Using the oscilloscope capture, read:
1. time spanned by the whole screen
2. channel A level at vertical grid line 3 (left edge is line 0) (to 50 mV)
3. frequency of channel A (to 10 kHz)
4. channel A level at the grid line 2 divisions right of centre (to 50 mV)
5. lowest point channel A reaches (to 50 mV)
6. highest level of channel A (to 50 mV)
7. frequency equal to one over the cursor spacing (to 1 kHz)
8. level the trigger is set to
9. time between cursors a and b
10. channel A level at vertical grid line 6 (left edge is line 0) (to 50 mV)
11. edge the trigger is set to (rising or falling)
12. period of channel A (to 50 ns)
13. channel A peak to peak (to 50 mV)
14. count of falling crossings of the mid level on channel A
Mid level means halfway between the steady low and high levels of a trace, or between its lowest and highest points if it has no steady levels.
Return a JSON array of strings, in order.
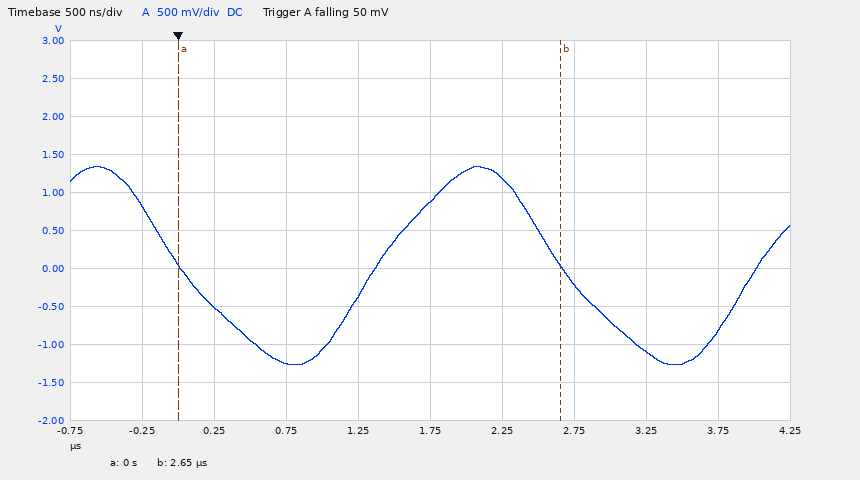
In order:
["5 µs", "-1.25 V", "380 kHz", "-200 mV", "-1.25 V", "1.35 V", "377 kHz", "50 mV", "2.65 µs", "1.20 V", "falling", "2.65 µs", "2.60 V", "2"]
